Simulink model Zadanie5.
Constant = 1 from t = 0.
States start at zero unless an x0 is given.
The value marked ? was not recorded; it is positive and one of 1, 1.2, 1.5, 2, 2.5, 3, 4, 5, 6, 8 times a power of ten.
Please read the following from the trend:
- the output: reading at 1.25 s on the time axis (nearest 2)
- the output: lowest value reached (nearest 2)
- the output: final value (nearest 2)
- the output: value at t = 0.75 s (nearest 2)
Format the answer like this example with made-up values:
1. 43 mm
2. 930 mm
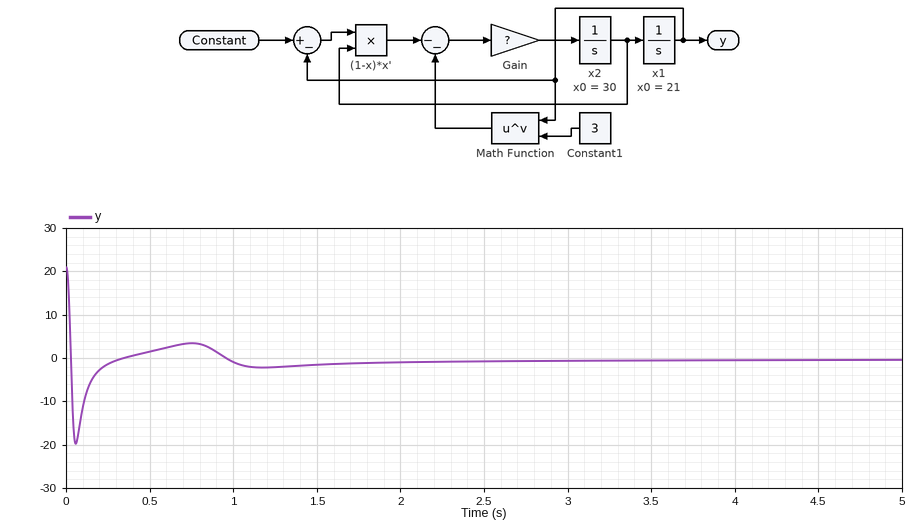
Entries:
1. -2
2. -20
3. 0
4. 4
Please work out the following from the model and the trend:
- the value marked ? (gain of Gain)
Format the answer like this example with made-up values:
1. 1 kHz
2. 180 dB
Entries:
1. 4
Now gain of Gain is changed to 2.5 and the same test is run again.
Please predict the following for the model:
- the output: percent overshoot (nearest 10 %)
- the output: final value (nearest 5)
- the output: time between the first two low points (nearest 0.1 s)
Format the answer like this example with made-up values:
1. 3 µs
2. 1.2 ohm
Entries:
1. 90 %
2. 0
3. 0.4 s
